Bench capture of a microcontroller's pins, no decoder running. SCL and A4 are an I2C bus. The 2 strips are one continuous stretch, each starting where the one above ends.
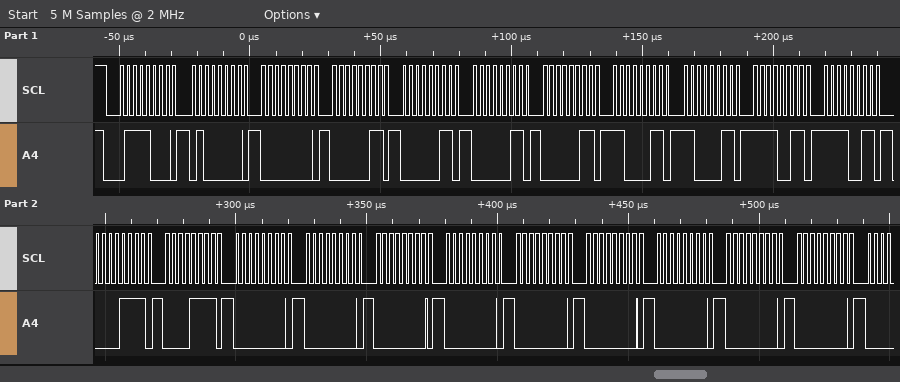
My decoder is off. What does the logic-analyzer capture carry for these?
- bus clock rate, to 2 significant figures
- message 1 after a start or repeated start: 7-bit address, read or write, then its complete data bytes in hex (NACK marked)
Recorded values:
400 kHz
0x3C write: 40 00 03 03 03 03 C3 C3 F3 F3 0F 0F 00 00 00 00 00 00 00 00 00
